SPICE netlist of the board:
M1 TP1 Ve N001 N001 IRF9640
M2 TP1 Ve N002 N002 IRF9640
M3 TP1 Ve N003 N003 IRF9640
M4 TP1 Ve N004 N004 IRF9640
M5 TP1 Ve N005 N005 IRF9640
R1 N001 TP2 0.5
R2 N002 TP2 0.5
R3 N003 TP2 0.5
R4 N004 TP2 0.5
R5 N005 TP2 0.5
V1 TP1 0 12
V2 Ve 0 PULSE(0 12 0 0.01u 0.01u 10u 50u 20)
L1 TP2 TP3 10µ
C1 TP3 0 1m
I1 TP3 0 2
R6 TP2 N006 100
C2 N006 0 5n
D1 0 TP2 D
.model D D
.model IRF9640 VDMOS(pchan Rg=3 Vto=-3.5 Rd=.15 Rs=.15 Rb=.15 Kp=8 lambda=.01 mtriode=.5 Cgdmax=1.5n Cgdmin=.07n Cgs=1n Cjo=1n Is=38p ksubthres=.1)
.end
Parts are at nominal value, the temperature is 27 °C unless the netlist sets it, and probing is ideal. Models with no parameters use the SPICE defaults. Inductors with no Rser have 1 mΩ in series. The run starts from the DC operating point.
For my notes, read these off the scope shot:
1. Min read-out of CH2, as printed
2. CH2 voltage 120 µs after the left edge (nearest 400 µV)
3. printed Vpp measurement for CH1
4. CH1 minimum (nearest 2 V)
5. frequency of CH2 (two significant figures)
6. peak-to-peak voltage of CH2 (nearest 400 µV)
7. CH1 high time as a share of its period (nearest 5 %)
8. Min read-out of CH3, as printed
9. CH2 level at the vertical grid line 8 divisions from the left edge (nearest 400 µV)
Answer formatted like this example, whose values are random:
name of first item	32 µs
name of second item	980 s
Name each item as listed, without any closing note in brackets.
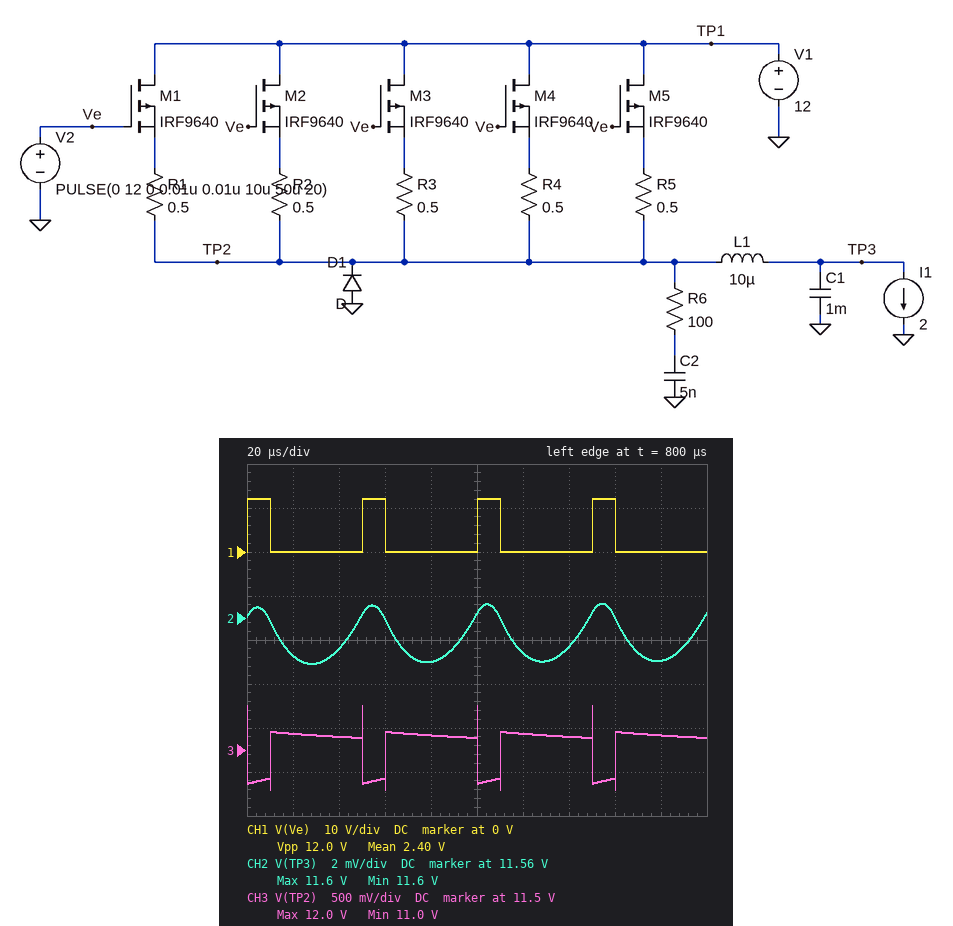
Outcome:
Min read-out of CH2, as printed	11.6 V
CH2 voltage 120 µs after the left edge	11.5604 V
printed Vpp measurement for CH1	12.0 V
CH1 minimum	0 V
frequency of CH2	20 kHz
peak-to-peak voltage of CH2	2.8 mV
CH1 high time as a share of its period	20 %
Min read-out of CH3, as printed	11.0 V
CH2 level at the vertical grid line 8 divisions from the left edge	11.5620 V
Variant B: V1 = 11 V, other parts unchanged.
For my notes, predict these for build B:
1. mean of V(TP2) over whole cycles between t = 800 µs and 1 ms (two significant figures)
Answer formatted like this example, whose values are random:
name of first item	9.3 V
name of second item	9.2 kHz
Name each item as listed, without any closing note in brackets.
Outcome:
mean of V(TP2) over whole cycles between t = 800 µs and 1 ms	11 V
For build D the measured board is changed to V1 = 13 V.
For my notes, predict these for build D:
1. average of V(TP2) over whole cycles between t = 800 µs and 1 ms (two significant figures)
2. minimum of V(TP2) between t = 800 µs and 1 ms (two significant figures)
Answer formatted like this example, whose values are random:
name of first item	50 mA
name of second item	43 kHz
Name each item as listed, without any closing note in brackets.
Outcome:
average of V(TP2) over whole cycles between t = 800 µs and 1 ms	13 V
minimum of V(TP2) between t = 800 µs and 1 ms	12 V
